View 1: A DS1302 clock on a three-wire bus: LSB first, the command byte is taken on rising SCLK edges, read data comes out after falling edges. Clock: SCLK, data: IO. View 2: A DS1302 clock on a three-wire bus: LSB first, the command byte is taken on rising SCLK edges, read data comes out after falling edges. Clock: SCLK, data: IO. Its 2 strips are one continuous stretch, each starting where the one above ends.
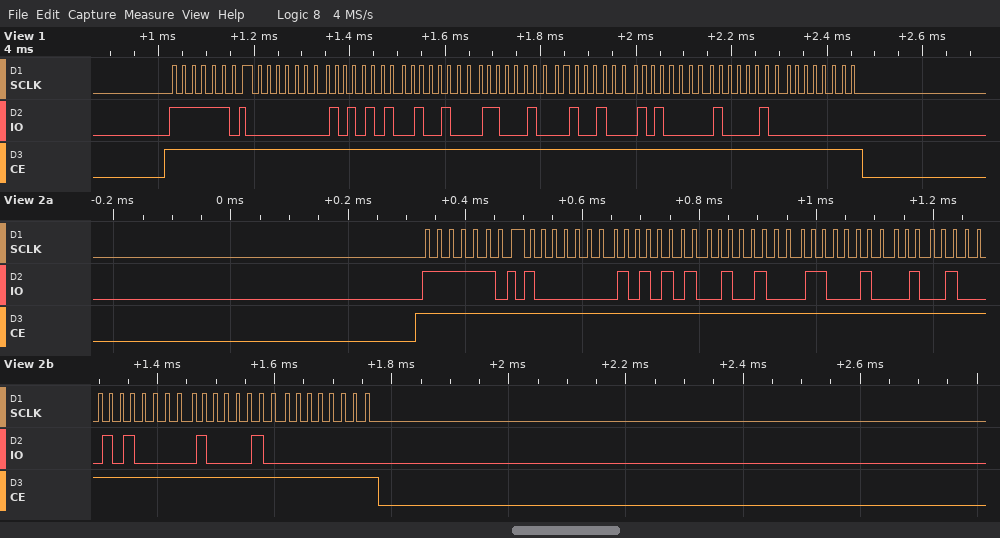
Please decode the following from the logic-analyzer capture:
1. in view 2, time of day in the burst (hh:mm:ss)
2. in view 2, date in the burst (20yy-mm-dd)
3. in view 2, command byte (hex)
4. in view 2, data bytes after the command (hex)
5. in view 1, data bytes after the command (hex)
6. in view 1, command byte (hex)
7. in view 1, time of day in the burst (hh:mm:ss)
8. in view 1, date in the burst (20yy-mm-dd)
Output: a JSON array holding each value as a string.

["12:55:01", "2021-12-23", "0xBF", "01 55 12 23 12 05 21 00", "00 55 12 23 12 05 21 00", "0xBF", "12:55:00", "2021-12-23"]
